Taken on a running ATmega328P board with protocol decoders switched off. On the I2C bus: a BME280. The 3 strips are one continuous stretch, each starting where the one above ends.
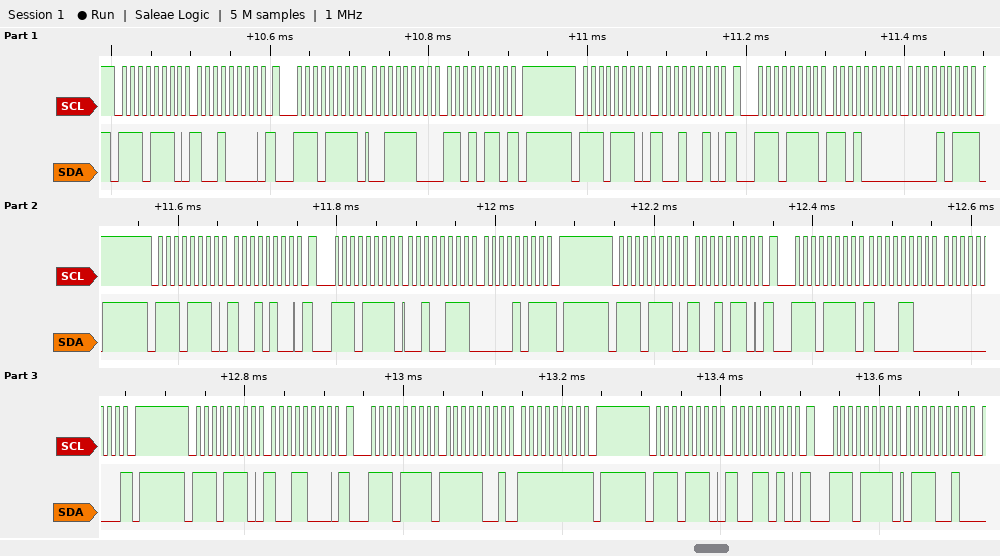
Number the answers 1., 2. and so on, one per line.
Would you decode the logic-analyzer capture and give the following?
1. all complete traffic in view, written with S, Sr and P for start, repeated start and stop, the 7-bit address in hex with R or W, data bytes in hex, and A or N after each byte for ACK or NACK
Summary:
1. S 77W A 90 A Sr 77R A 3C A D6 N P S 77W A 92 A Sr 77R A D0 A 0B N P S 77W A 94 A Sr 77R A 27 A 0B N P S 77W A 96 A Sr 77R A 8C A 00 N P S 77W A 98 A Sr 77R A F9 A FF N P S 77W A 9A A Sr 77R A 72 A
